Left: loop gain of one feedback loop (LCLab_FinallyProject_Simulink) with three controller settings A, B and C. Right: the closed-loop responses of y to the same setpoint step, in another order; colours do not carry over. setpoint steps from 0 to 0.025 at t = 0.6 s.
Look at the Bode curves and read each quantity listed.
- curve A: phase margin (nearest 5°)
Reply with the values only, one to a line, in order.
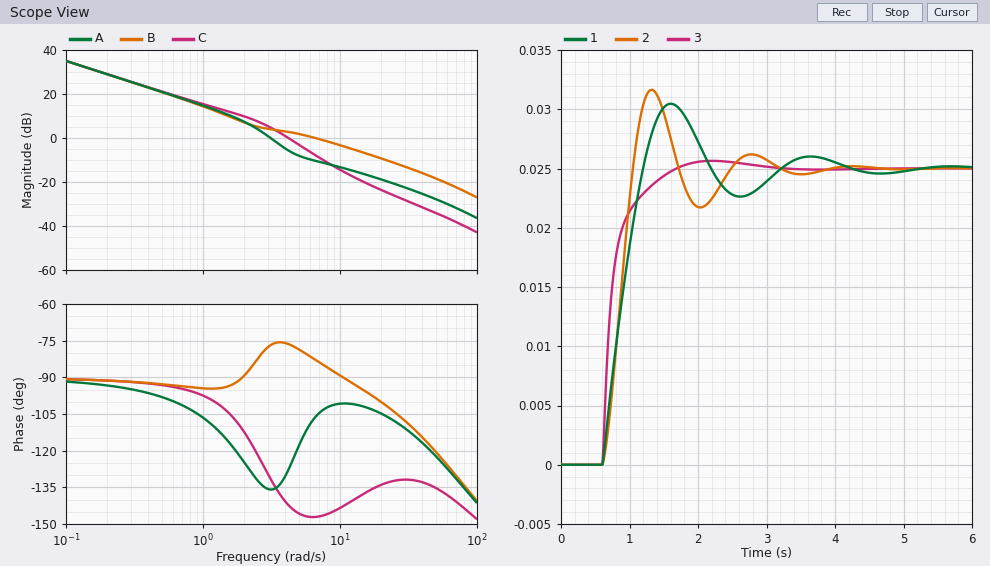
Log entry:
45°
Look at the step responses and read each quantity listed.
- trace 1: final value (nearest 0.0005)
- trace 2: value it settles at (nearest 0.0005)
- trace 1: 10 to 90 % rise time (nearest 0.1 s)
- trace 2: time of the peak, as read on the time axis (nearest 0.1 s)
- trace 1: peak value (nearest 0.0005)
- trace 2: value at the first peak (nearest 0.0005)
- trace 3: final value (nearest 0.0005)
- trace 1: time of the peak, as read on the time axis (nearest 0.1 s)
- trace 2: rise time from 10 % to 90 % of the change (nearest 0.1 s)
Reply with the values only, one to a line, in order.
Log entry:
0.0250
0.0250
0.5 s
1.3 s
0.0305
0.0315
0.0250
1.6 s
0.3 s
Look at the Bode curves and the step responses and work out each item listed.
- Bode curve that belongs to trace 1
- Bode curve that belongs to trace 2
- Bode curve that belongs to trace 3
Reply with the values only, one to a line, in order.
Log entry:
A
C
B
